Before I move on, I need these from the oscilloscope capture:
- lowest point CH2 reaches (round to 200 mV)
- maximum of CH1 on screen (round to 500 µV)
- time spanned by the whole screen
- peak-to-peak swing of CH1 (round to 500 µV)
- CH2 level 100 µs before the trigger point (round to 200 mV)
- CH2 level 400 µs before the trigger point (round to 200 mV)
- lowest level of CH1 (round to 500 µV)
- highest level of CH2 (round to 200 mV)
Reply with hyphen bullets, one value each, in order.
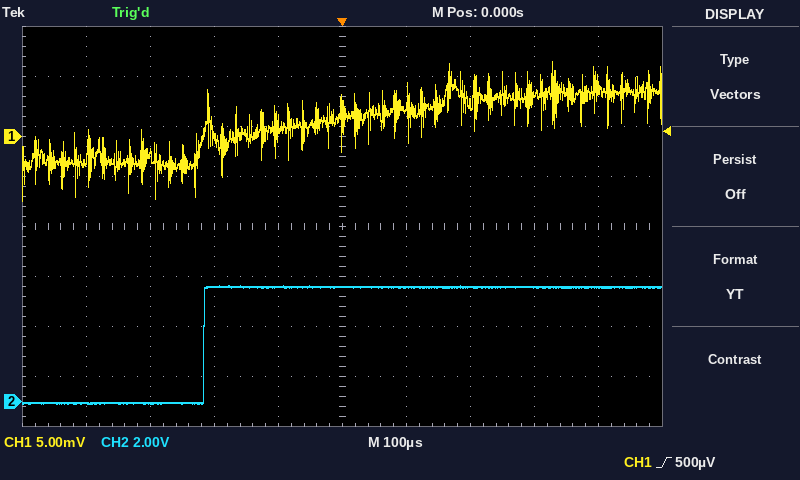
- 0.0 V
- 7.5 mV
- 1 ms
- 14.0 mV
- 4.6 V
- 0.0 V
- -6.5 mV
- 4.6 V
